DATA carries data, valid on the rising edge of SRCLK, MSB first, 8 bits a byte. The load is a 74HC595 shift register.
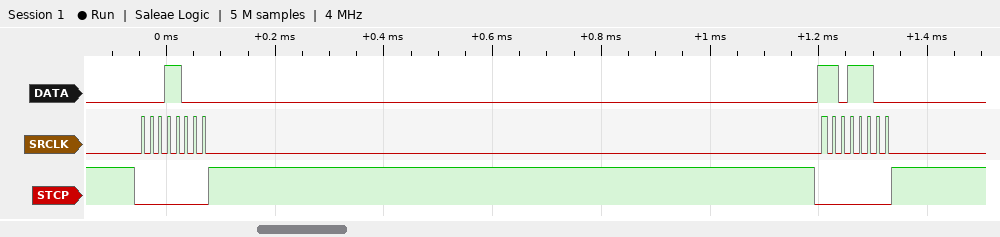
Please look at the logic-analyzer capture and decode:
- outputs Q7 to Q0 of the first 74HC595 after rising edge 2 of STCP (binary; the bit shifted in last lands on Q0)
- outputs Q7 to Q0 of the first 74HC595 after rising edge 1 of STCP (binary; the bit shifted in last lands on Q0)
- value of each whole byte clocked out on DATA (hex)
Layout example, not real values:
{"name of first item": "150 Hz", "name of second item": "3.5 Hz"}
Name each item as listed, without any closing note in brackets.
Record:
{"outputs Q7 to Q0 of the first 74HC595 after rising edge 2 of STCP": "11011100", "outputs Q7 to Q0 of the first 74HC595 after rising edge 1 of STCP": "00011000", "value of each whole byte clocked out on DATA": "18 DC"}
